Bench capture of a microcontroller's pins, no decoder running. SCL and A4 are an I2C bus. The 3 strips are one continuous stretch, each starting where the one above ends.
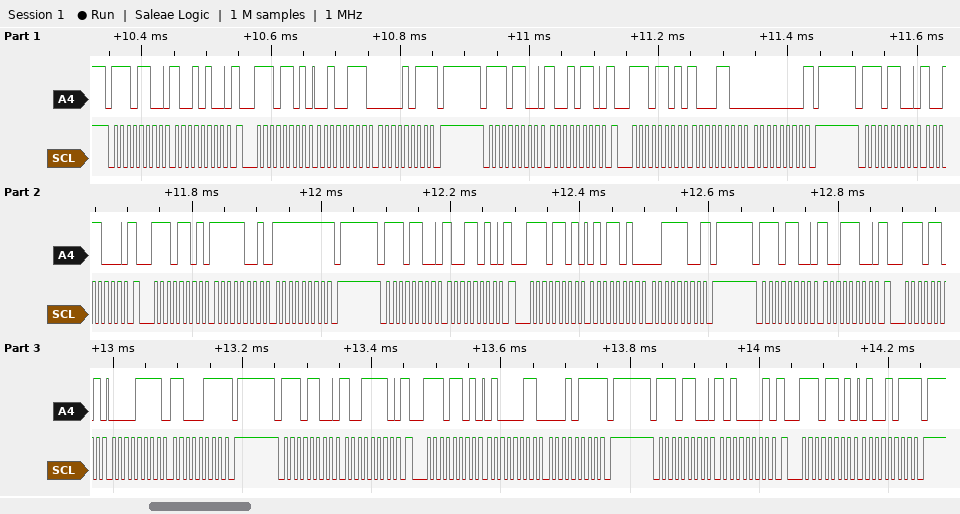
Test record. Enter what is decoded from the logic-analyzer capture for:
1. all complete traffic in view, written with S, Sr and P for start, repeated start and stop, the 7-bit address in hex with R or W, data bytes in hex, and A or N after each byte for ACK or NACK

S 76W A 94 A Sr 76R A 27 A 0B N P S 76W A 96 A Sr 76R A 8C A 00 N P S 76W A 98 A Sr 76R A F9 A FF N P S 76W A 9A A Sr 76R A 5A A 3C N P S 76W A 9C A Sr 76R A 0F A C7 N P S 76W A 9E A Sr 76R A 43 A 17 N P S 76W A A1 A Sr 76R A 4B N P
